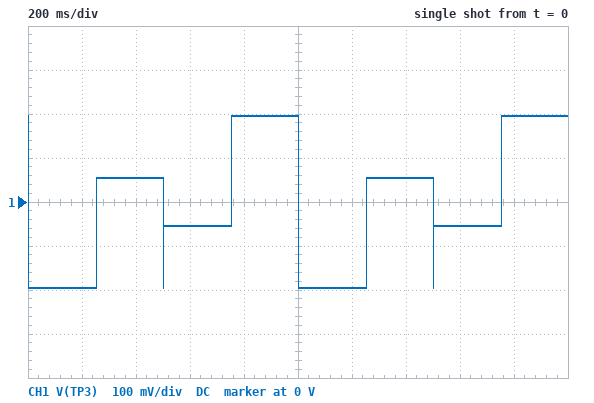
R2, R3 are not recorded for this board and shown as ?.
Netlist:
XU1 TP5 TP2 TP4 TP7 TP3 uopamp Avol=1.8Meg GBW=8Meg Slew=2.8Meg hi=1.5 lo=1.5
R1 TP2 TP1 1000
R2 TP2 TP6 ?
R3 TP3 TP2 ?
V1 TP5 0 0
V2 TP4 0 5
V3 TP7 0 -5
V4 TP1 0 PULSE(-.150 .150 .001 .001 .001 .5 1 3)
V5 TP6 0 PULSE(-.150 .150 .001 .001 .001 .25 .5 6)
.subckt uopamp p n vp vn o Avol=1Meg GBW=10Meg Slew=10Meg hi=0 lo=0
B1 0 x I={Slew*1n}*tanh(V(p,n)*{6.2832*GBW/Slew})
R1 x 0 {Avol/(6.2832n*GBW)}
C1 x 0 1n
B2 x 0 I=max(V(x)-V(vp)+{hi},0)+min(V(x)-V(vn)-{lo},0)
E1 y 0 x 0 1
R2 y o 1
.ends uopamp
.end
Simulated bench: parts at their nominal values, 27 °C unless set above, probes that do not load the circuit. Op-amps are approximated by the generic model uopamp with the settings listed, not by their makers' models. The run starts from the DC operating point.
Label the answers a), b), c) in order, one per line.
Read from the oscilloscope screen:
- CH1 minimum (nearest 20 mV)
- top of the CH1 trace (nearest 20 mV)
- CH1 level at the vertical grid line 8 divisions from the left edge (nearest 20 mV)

a) -200 mV
b) 200 mV
c) -60 mV
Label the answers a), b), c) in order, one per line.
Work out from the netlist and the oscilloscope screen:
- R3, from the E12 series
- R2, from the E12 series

a) 470 Ω
b) 560 Ω
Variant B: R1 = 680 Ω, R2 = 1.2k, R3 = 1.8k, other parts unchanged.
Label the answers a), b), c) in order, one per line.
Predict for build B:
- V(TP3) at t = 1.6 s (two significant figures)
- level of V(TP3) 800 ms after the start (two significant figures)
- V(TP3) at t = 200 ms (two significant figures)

a) 170 mV
b) 620 mV
c) -620 mV
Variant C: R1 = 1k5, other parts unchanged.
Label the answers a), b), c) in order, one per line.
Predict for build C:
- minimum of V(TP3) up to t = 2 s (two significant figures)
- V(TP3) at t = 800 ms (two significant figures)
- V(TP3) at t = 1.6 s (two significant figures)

a) -170 mV
b) 170 mV
c) -79 mV
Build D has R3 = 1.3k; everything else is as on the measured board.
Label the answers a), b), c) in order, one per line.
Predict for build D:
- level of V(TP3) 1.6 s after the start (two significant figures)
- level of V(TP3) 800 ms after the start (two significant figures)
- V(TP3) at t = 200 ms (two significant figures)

a) -150 mV
b) 540 mV
c) -540 mV
